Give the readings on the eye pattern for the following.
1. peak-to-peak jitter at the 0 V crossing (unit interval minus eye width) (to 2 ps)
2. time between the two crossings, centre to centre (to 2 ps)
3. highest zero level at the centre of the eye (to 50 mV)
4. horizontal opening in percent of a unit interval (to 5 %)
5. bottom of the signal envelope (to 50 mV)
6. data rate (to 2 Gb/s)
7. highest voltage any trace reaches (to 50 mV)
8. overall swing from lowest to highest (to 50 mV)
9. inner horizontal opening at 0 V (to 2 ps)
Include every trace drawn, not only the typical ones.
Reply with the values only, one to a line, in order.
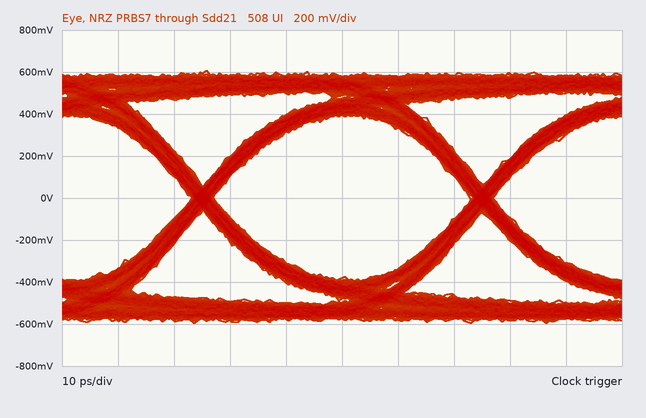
4 ps
50 ps
-400 mV
90 %
-600 mV
20 Gb/s
600 mV
1.20 V
46 ps
